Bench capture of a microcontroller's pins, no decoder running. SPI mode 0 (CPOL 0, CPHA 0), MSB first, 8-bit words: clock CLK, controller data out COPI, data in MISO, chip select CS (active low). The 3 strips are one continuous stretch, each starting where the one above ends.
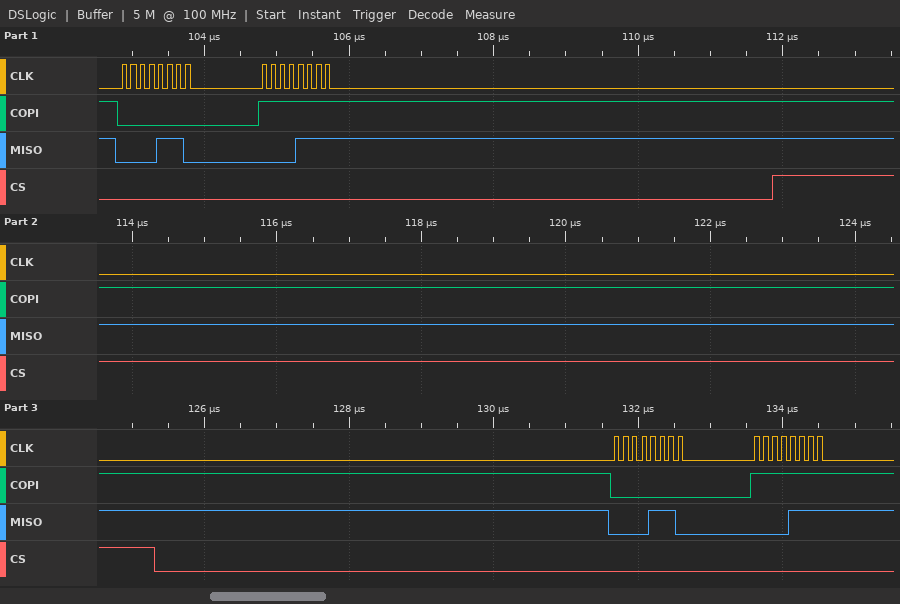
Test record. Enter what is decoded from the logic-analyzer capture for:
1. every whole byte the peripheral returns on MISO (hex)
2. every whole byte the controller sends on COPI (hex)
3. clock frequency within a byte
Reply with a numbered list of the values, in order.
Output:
1. 0E 0F 0E 0F
2. 00 FF 00 FF
3. 8 MHz
